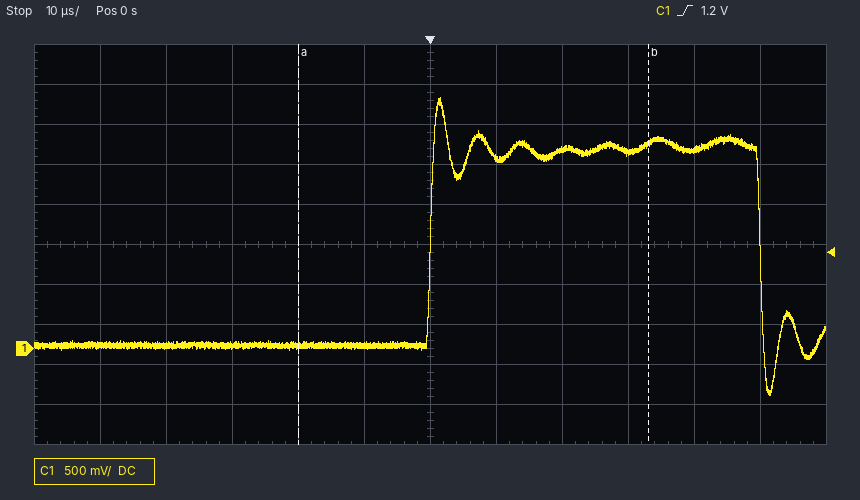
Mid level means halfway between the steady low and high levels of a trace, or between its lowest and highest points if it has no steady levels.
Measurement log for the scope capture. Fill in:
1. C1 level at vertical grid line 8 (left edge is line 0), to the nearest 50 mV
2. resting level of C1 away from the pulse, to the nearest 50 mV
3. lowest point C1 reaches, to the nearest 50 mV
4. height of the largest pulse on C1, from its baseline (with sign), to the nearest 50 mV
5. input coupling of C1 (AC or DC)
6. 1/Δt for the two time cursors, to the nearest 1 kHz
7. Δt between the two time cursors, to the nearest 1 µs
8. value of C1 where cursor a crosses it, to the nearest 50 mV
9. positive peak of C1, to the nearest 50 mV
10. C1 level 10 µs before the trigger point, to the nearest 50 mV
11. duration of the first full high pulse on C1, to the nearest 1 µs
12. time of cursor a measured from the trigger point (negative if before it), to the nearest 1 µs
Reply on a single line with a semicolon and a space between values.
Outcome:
2.50 V; 50 mV; -600 mV; +3.10 V; DC; 19 kHz; 53 µs; 50 mV; 3.15 V; 50 mV; 50 µs; -20 µs
